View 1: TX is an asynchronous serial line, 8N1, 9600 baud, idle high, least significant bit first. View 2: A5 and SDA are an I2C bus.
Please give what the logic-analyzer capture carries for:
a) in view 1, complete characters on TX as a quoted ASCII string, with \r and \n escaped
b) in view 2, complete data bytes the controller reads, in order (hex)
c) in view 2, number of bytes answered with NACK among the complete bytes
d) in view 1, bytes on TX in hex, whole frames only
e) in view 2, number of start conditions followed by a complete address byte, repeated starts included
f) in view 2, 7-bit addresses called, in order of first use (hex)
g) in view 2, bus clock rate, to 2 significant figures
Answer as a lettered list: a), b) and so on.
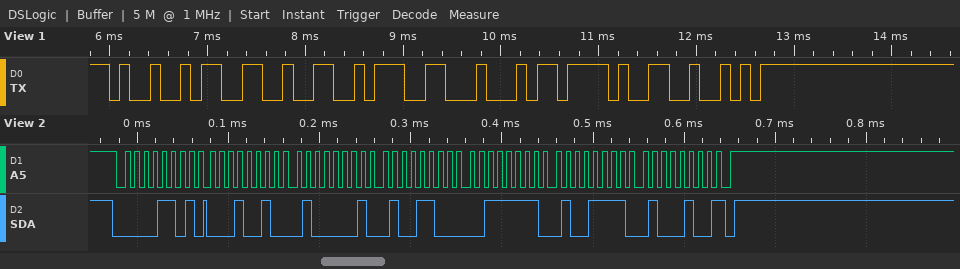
a) "I&:D/R"
b) 12 41 4C 3F 4F 44
c) 1
d) 49 26 3A 44 2F 52
e) 1
f) 0x06
g) 100 kHz
